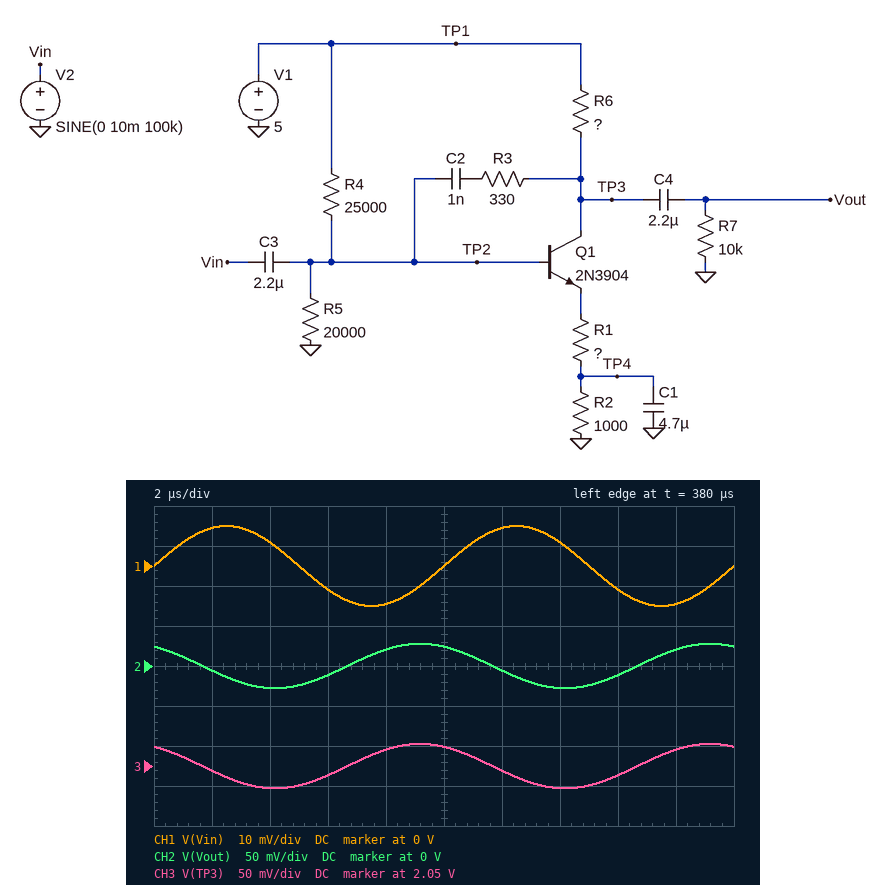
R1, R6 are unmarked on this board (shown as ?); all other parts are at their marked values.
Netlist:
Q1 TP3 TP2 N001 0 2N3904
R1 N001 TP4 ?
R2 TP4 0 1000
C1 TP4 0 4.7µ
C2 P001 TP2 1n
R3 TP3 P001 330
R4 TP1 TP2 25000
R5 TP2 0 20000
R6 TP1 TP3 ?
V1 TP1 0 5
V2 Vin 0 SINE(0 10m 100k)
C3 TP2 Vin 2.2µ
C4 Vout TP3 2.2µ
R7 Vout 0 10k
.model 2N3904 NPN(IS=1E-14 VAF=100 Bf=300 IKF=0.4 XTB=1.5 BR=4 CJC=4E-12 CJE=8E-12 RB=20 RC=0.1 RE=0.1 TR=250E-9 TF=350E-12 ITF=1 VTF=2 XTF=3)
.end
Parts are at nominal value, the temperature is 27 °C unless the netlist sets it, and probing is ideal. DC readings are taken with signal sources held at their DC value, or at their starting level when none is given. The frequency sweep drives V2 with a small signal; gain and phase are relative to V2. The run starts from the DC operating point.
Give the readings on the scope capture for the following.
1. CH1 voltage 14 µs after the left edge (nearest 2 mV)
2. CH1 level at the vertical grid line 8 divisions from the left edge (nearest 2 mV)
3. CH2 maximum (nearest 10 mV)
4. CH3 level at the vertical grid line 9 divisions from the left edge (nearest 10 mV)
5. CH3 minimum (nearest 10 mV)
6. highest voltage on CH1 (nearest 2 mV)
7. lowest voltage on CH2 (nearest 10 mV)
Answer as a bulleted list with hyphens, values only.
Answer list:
- 6 mV
- -6 mV
- 30 mV
- 2.07 V
- 2.02 V
- 10 mV
- -30 mV
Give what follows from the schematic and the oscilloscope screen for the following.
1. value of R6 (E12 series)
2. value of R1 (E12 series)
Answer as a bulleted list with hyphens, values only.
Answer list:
- 2.7 kΩ
- 390 Ω
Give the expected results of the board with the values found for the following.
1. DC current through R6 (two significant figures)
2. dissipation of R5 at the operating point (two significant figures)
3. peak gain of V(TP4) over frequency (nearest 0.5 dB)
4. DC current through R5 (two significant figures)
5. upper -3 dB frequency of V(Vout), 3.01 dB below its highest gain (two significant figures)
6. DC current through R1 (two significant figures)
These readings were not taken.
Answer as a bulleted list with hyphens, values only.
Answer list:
- 1.1 mA
- 240 µW
- -3.5 dB
- 110 µA
- 65 kHz
- 1.1 mA
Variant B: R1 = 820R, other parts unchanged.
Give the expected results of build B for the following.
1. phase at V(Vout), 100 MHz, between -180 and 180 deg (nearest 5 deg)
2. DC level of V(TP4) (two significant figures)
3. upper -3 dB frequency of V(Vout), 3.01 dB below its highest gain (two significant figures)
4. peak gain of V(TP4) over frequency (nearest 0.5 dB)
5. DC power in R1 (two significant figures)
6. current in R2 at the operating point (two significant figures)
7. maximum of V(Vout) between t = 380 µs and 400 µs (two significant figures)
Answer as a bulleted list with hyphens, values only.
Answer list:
- 20 deg
- 850 mV
- 68 kHz
- -6.0 dB
- 590 µW
- 850 µA
- 14 mV
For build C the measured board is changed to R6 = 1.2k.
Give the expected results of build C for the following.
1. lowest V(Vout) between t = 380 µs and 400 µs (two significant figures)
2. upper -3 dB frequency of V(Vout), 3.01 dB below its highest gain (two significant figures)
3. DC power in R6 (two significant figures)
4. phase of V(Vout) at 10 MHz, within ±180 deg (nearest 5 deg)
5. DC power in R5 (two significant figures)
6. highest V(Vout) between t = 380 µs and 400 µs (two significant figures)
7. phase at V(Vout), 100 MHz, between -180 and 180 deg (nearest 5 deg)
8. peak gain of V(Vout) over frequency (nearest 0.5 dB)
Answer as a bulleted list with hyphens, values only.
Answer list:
- -19 mV
- 110 kHz
- 1.4 mW
- 30 deg
- 240 µW
- 19 mV
- 45 deg
- 8.0 dB
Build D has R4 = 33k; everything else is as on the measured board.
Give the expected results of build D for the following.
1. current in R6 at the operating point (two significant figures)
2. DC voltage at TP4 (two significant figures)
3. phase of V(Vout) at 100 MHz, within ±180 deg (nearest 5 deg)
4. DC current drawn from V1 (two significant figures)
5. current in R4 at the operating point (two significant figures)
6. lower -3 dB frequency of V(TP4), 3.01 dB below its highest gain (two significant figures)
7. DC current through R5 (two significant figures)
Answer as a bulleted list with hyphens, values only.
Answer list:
- 860 µA
- 860 mV
- 40 deg
- 960 µA
- 95 µA
- 5.4 Hz
- 93 µA
